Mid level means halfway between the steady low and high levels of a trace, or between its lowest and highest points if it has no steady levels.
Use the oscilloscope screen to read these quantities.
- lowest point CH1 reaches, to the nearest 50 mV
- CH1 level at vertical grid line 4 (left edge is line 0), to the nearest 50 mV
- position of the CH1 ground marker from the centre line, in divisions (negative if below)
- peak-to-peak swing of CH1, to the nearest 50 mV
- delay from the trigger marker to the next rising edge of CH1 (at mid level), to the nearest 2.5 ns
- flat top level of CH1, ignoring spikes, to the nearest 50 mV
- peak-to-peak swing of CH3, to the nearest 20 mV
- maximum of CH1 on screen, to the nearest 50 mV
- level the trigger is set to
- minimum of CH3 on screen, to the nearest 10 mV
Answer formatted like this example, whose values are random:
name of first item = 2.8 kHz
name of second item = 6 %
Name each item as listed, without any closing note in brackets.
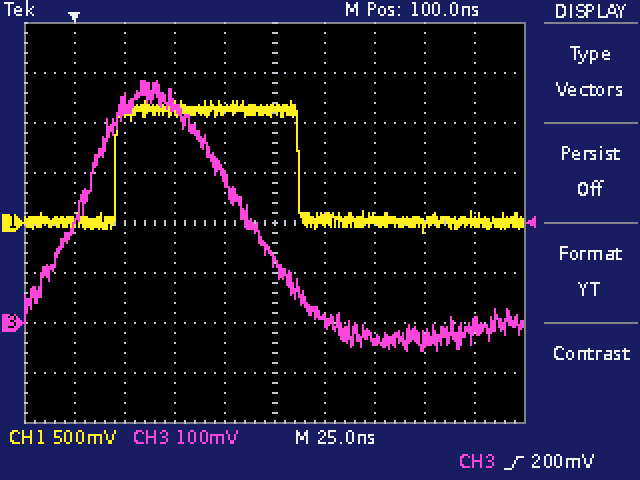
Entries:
lowest point CH1 reaches, to the nearest 50 mV = -100 mV
CH1 level at vertical grid line 4 (left edge is line 0), to the nearest 50 mV = 1.15 V
position of the CH1 ground marker from the centre line, in divisions = 0.0 div
peak-to-peak swing of CH1, to the nearest 50 mV = 1.30 V
delay from the trigger marker to the next rising edge of CH1 (at mid level), to the nearest 2.5 ns = 20.0 ns
flat top level of CH1, ignoring spikes, to the nearest 50 mV = 1.15 V
peak-to-peak swing of CH3, to the nearest 20 mV = 540 mV
maximum of CH1 on screen, to the nearest 50 mV = 1.20 V
level the trigger is set to = 200 mV
minimum of CH3 on screen, to the nearest 10 mV = -60 mV
